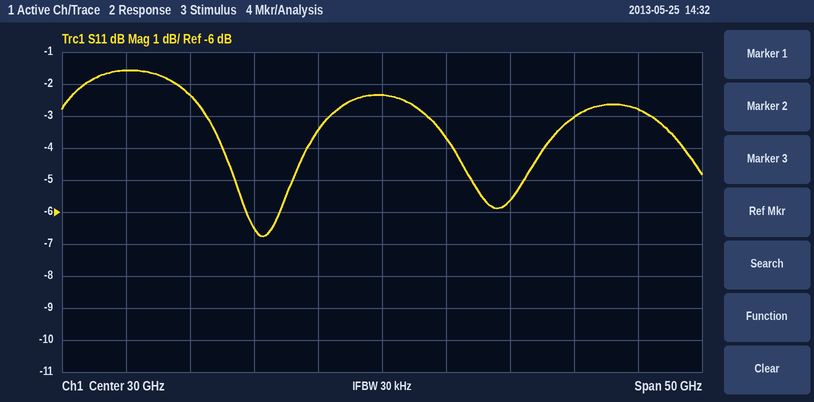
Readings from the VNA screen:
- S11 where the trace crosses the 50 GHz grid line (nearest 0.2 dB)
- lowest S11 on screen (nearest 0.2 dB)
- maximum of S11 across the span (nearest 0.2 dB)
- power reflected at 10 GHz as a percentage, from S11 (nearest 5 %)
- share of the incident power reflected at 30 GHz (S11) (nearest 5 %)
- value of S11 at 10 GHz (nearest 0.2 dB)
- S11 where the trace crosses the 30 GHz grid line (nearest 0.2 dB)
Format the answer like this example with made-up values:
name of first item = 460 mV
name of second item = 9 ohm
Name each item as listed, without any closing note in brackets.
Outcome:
S11 where the trace crosses the 50 GHz grid line = -2.8 dB
lowest S11 on screen = -6.8 dB
maximum of S11 across the span = -1.6 dB
power reflected at 10 GHz as a percentage, from S11 = 70 %
share of the incident power reflected at 30 GHz (S11) = 60 %
value of S11 at 10 GHz = -1.6 dB
S11 where the trace crosses the 30 GHz grid line = -2.4 dB
